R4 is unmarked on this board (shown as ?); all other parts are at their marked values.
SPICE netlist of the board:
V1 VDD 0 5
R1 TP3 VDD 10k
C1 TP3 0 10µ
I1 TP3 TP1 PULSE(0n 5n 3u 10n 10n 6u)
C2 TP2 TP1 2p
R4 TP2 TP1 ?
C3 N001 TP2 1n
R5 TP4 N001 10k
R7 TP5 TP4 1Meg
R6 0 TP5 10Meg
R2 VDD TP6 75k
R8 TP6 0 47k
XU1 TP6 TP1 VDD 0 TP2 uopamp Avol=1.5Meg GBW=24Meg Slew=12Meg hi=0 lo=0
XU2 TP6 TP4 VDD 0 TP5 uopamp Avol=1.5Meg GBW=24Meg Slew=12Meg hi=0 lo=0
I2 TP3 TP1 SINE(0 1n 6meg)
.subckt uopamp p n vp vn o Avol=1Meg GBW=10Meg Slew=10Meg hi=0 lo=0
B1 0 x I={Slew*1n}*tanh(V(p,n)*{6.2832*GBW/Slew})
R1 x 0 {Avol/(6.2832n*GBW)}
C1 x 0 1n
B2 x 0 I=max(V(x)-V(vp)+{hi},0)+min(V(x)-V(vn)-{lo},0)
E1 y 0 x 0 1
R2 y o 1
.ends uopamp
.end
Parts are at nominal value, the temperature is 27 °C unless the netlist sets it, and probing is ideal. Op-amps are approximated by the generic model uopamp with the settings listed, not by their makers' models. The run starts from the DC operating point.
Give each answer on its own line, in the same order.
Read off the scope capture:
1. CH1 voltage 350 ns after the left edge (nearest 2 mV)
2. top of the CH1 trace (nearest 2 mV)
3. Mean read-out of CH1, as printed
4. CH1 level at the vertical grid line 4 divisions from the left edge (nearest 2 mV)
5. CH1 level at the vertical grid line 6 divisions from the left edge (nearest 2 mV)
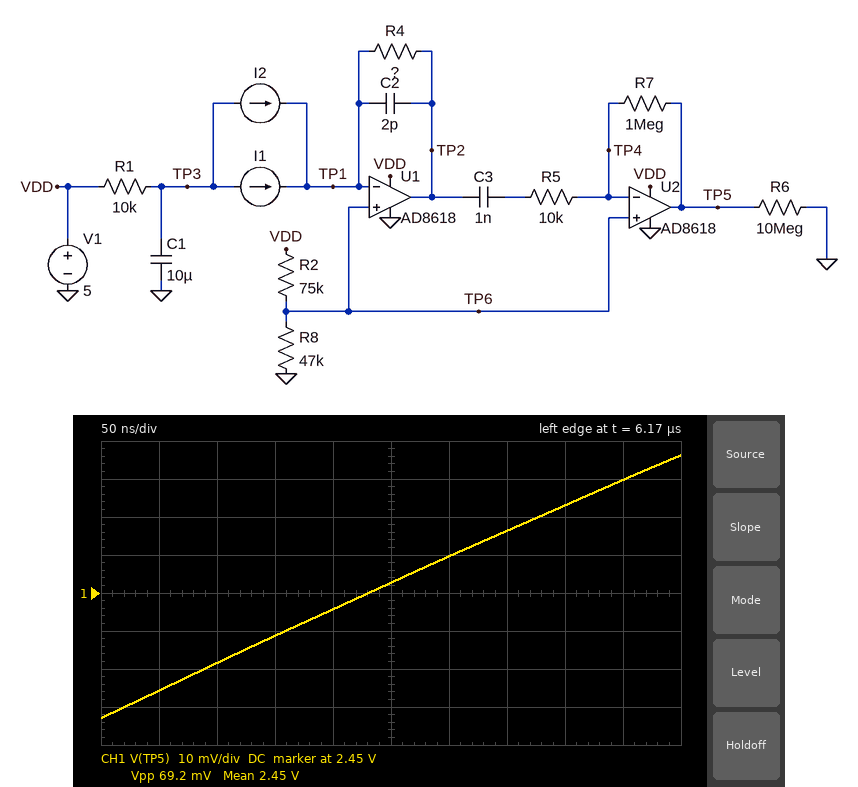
2.466 V
2.486 V
2.45 V
2.446 V
2.460 V
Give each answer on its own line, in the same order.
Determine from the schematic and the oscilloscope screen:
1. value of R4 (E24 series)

4.3 MΩ
